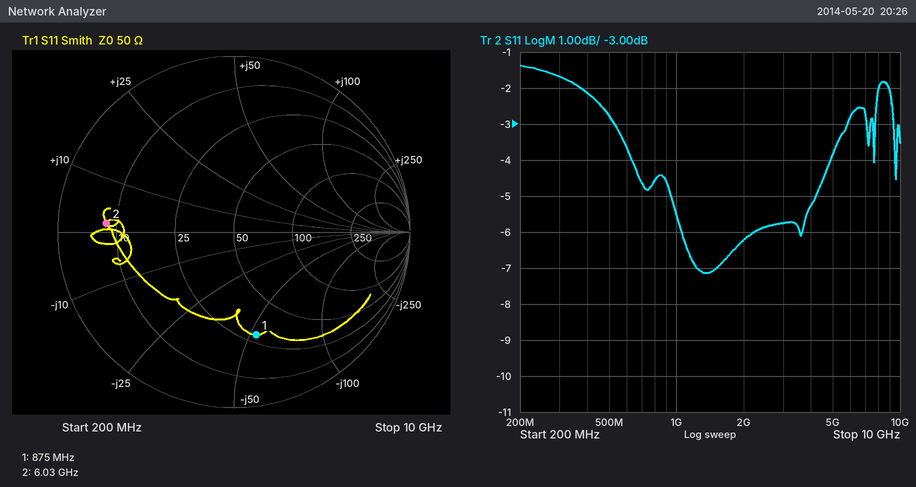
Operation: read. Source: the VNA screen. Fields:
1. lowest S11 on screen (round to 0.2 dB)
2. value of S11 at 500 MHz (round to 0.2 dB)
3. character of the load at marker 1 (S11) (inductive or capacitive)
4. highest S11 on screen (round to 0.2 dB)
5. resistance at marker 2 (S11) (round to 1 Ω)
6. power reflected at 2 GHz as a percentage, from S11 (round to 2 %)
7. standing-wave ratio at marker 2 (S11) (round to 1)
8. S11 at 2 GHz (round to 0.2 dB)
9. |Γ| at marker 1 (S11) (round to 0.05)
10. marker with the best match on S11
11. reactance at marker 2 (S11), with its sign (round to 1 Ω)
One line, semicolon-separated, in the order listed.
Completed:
-7.2 dB; -2.8 dB; capacitive; -1.4 dB; 8 Ω; 24 %; 6; -6.2 dB; 0.60; marker 1; +2 Ω
